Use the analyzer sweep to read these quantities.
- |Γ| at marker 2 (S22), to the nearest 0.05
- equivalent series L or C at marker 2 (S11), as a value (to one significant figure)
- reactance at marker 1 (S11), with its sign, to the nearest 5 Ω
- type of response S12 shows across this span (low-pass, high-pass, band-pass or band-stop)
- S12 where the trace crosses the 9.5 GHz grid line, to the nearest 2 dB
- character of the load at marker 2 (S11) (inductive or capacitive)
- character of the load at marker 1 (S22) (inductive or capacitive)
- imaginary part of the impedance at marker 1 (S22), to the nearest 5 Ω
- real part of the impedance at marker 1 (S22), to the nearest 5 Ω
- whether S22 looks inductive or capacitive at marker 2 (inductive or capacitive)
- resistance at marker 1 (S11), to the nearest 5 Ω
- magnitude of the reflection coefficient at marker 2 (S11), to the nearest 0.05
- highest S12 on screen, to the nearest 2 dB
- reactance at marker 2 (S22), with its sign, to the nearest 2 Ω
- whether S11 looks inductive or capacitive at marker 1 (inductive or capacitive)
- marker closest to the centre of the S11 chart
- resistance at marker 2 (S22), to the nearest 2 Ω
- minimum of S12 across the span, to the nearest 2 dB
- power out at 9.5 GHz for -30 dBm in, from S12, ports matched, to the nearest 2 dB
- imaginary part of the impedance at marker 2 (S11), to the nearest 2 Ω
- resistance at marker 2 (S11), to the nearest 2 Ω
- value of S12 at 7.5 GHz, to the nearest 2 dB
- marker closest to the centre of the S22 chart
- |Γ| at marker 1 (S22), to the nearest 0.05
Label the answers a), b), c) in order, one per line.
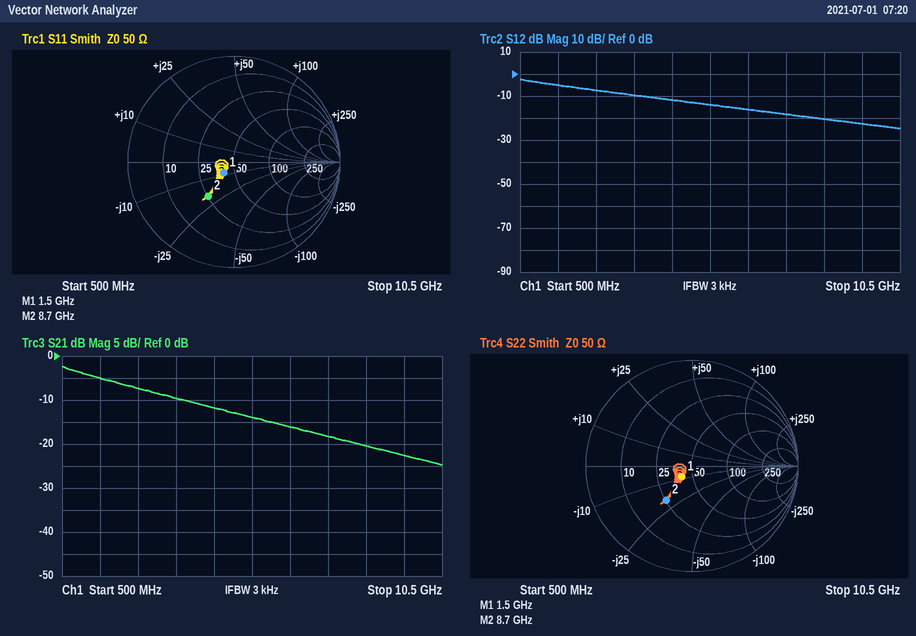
a) 0.40
b) 900 fF
c) -10 Ω
d) low-pass
e) -22 dB
f) capacitive
g) capacitive
h) -10 Ω
i) 40 Ω
j) capacitive
k) 40 Ω
l) 0.40
m) -2 dB
n) -20 Ω
o) capacitive
p) marker 1
q) 26 Ω
r) -24 dB
s) -52 dBm
t) -20 Ω
u) 26 Ω
v) -18 dB
w) marker 1
x) 0.15
